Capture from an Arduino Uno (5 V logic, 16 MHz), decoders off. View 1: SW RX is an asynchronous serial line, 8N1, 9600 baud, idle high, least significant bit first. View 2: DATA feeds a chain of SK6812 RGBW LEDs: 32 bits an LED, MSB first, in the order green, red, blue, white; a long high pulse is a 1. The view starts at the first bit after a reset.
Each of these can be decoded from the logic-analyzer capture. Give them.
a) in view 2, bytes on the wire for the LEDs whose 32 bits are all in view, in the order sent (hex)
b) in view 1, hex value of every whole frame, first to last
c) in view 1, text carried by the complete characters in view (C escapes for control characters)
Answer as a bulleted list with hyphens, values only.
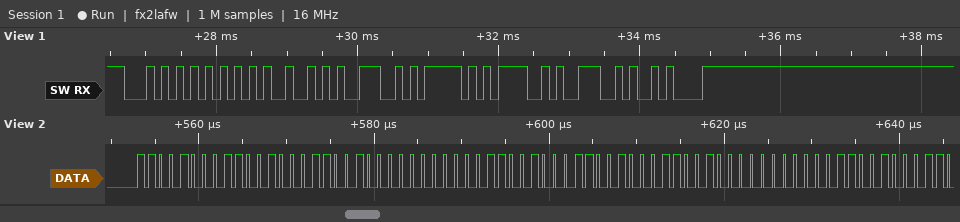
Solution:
- C8 C8 C8 00 C8 C8 C8 00
- 54 55 52 4E 5F 4F 4E 0A
- "TURN_ON\n"
